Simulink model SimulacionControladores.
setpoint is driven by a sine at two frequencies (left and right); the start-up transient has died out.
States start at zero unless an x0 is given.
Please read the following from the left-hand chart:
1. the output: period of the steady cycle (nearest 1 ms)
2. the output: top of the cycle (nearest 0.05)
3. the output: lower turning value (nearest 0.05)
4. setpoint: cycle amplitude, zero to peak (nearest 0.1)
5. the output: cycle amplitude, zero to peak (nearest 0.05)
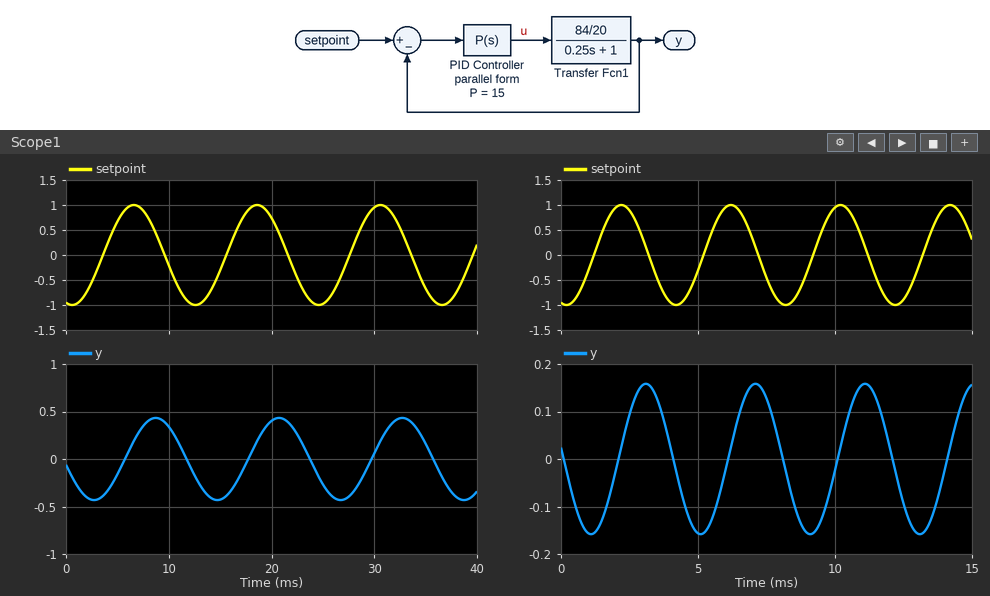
12 ms
0.45
-0.45
1.0
0.45
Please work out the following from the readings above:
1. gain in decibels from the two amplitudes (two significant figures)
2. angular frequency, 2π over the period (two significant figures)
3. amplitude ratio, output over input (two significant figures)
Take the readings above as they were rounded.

-6.9 dB
0.52 rad/ms
0.45
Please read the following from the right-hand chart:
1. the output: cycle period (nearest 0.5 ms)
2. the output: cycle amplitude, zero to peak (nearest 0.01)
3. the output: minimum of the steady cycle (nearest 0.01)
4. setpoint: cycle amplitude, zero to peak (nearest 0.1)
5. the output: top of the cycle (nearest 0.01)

4.0 ms
0.16
-0.16
1.0
0.16
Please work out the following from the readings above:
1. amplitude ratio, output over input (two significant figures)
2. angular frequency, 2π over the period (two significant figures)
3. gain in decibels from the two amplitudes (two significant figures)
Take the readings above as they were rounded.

0.16
1.6 rad/ms
-16 dB
